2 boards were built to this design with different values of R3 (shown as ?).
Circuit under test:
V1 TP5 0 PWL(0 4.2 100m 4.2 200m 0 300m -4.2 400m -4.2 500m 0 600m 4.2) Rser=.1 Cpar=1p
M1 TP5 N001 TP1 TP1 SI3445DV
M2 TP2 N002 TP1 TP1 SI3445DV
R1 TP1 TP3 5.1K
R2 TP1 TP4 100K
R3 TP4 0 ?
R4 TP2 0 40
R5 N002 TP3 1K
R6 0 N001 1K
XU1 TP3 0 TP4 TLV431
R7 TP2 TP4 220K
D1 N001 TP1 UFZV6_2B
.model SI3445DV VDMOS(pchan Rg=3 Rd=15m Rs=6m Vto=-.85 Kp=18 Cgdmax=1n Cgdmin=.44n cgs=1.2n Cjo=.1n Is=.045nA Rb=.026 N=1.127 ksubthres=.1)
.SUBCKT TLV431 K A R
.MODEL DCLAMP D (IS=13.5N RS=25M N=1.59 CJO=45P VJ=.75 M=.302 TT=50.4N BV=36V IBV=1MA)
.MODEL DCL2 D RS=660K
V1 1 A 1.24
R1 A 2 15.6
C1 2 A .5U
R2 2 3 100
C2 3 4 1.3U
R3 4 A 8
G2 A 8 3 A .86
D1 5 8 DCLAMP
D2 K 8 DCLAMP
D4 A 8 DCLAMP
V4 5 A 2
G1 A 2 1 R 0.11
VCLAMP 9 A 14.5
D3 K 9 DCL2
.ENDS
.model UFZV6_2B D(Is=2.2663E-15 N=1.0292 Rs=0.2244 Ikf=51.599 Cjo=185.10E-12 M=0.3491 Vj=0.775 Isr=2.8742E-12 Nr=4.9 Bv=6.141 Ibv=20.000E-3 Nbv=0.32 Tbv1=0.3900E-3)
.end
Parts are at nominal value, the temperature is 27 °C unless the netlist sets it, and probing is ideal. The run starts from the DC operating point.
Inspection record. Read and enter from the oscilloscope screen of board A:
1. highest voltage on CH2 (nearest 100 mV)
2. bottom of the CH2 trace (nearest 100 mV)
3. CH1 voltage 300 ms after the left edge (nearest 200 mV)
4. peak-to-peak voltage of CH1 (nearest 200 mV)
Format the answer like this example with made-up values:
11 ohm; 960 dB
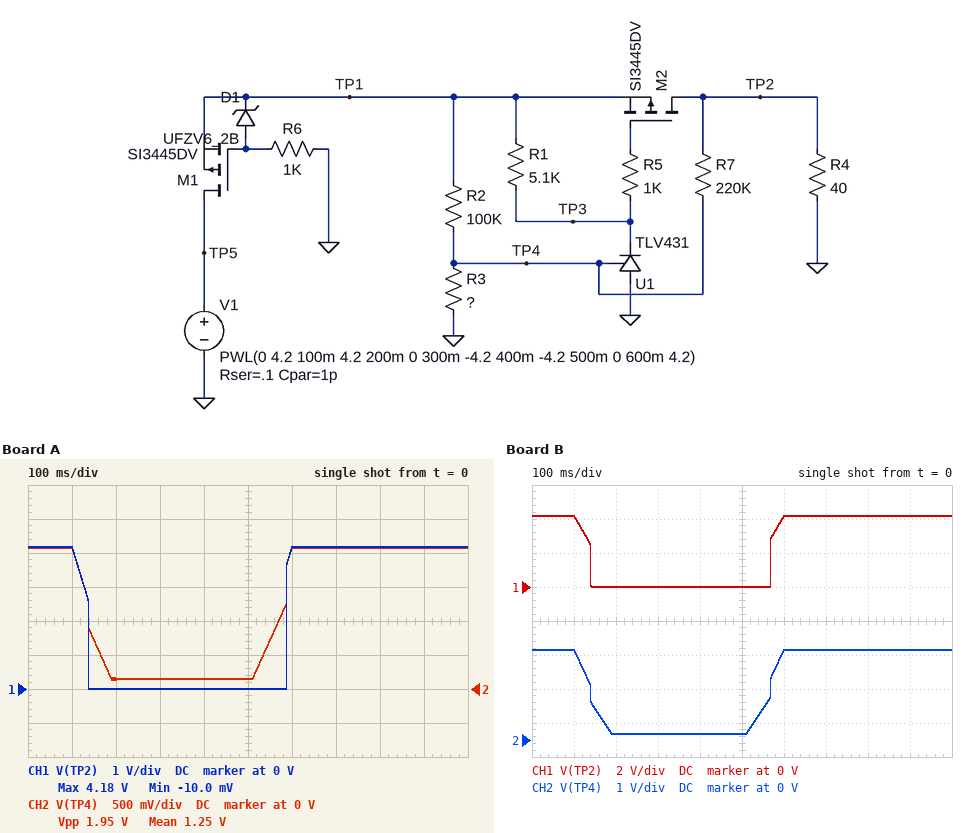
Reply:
2.1 V; 100 mV; 0 V; 4.2 V
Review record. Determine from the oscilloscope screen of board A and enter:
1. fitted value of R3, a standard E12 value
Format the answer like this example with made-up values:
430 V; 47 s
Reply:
68 kΩ
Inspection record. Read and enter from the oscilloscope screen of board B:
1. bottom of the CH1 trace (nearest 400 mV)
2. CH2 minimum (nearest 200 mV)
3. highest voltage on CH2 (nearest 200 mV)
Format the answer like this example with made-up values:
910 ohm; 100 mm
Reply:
0 V; 200 mV; 2.6 V
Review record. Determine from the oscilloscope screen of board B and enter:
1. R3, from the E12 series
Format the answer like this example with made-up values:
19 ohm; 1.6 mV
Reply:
120 kΩ
